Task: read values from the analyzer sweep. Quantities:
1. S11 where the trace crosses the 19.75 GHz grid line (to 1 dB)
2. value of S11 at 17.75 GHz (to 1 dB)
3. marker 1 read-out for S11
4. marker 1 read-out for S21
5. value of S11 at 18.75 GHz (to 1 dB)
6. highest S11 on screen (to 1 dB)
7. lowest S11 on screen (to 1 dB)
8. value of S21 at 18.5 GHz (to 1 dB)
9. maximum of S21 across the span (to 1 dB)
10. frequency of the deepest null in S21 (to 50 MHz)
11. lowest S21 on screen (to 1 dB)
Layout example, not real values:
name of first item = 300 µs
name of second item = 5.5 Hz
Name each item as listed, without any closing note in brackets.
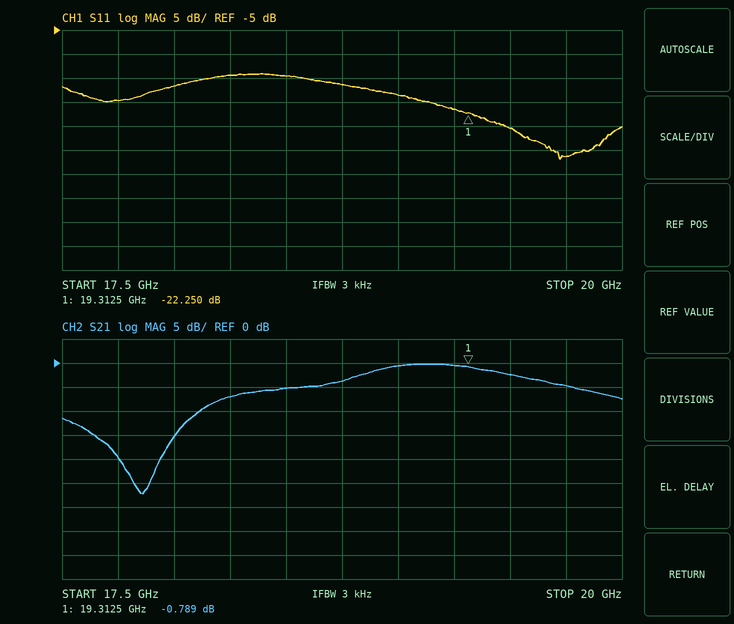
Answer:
S11 where the trace crosses the 19.75 GHz grid line = -31 dB
value of S11 at 17.75 GHz = -20 dB
marker 1 read-out for S11 = -22.250 dB
marker 1 read-out for S21 = -0.789 dB
value of S11 at 18.75 GHz = -16 dB
highest S11 on screen = -14 dB
lowest S11 on screen = -32 dB
value of S21 at 18.5 GHz = -5 dB
maximum of S21 across the span = 0 dB
frequency of the deepest null in S21 = 17.85 GHz
lowest S21 on screen = -27 dB
